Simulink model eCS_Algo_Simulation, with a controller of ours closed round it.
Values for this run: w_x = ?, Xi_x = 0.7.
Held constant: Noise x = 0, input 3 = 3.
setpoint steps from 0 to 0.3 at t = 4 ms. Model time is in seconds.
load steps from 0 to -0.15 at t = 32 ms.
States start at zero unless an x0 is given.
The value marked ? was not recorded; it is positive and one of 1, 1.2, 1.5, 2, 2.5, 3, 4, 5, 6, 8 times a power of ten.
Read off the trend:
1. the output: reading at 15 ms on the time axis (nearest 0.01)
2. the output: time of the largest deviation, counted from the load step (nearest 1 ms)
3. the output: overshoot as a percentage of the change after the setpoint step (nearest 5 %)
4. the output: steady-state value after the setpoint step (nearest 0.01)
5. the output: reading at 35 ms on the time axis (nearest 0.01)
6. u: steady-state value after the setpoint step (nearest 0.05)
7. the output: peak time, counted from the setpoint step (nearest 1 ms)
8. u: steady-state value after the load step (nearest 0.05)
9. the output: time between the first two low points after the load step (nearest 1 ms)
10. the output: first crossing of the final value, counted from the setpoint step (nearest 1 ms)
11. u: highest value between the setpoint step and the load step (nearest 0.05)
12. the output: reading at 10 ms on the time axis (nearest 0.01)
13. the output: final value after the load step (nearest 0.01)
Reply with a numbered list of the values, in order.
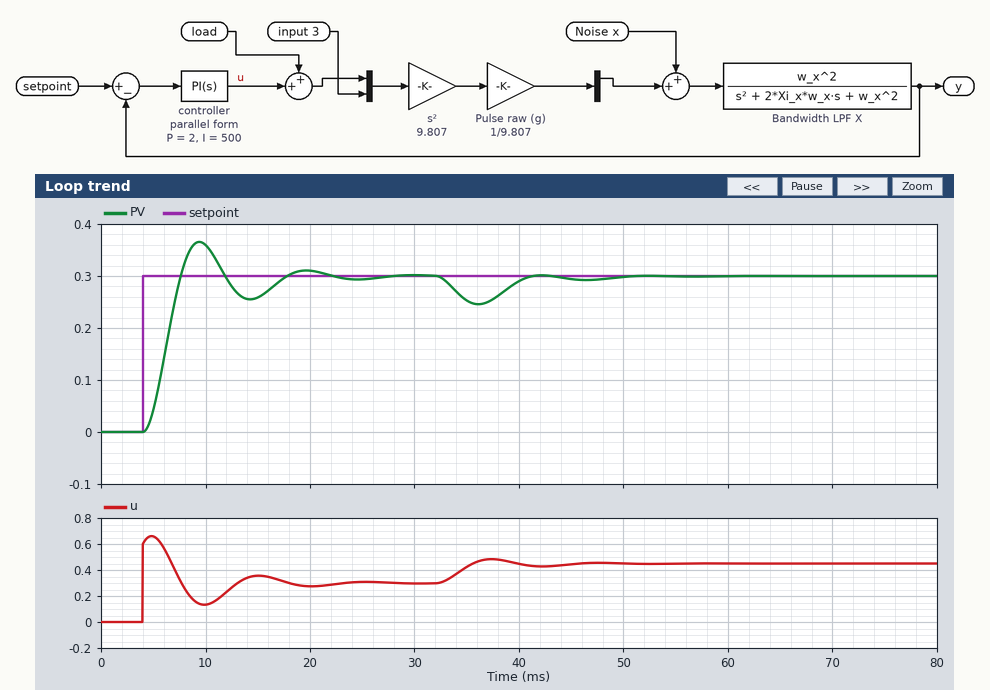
1. 0.26
2. 4 ms
3. 20 %
4. 0.30
5. 0.25
6. 0.30
7. 5 ms
8. 0.45
9. 10 ms
10. 4 ms
11. 0.65
12. 0.36
13. 0.30
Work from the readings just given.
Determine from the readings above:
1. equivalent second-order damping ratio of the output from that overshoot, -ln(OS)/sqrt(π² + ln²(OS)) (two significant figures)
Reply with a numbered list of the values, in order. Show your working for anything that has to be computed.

1. ln(0.2) = -1.609; 1.609 / sqrt(9.870 + 2.590) = 0.46
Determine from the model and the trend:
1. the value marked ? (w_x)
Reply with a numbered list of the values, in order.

1. 400
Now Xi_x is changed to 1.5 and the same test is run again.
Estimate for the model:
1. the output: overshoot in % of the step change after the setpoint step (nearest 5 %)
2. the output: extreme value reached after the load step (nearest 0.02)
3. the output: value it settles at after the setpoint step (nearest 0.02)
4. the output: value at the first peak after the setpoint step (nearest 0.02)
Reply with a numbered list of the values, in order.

1. 10 %
2. 0.26
3. 0.30
4. 0.34
